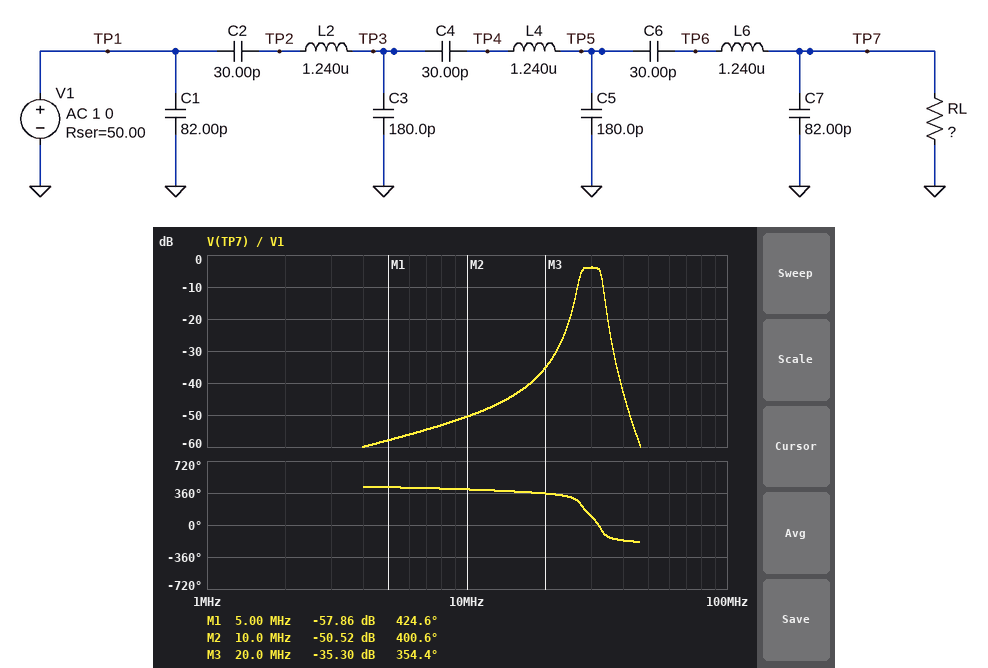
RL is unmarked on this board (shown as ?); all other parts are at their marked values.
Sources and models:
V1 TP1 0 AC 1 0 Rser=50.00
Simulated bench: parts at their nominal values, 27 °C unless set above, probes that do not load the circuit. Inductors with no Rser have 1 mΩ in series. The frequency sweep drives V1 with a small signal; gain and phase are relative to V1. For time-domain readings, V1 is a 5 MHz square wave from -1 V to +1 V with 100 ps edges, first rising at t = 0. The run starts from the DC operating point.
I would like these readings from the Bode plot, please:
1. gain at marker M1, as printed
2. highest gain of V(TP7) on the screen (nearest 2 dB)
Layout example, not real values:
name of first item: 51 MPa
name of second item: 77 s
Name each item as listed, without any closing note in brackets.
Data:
gain at marker M1, as printed: -57.86 dB
highest gain of V(TP7) on the screen: -4 dB
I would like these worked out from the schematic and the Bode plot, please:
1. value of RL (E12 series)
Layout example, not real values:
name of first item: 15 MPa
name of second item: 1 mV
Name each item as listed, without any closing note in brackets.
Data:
value of RL: 82 Ω
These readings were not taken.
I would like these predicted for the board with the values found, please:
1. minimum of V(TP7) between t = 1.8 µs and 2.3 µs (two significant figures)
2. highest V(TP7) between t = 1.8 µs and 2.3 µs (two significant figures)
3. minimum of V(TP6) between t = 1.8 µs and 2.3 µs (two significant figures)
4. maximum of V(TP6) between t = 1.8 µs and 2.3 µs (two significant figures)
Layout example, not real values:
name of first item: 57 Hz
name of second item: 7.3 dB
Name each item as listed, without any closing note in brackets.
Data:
minimum of V(TP7) between t = 1.8 µs and 2.3 µs: -46 mV
highest V(TP7) between t = 1.8 µs and 2.3 µs: 46 mV
minimum of V(TP6) between t = 1.8 µs and 2.3 µs: -160 mV
maximum of V(TP6) between t = 1.8 µs and 2.3 µs: 160 mV
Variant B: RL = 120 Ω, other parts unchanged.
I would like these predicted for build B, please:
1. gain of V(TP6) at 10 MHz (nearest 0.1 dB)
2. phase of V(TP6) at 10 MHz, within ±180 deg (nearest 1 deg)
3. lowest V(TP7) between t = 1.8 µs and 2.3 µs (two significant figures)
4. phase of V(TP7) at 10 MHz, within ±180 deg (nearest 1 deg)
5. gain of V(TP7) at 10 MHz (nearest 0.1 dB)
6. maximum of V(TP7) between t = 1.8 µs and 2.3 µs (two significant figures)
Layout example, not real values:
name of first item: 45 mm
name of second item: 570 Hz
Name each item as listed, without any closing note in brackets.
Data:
gain of V(TP6) at 10 MHz: -49.4 dB
phase of V(TP6) at 10 MHz, within ±180 deg: 78 deg
lowest V(TP7) between t = 1.8 µs and 2.3 µs: -52 mV
phase of V(TP7) at 10 MHz, within ±180 deg: 30 deg
gain of V(TP7) at 10 MHz: -48.3 dB
maximum of V(TP7) between t = 1.8 µs and 2.3 µs: 52 mV
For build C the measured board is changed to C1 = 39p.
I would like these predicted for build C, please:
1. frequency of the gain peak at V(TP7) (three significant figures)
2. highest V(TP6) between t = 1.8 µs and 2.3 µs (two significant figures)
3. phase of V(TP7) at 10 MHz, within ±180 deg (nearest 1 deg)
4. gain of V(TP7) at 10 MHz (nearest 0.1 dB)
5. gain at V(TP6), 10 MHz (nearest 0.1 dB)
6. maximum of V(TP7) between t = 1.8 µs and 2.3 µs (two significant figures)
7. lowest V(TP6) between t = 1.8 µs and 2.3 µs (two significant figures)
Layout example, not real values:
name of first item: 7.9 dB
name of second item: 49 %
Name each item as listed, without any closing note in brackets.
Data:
frequency of the gain peak at V(TP7): 29.5 MHz
highest V(TP6) between t = 1.8 µs and 2.3 µs: 170 mV
phase of V(TP7) at 10 MHz, within ±180 deg: 48 deg
gain of V(TP7) at 10 MHz: -50.2 dB
gain at V(TP6), 10 MHz: -49.2 dB
maximum of V(TP7) between t = 1.8 µs and 2.3 µs: 52 mV
lowest V(TP6) between t = 1.8 µs and 2.3 µs: -170 mV
